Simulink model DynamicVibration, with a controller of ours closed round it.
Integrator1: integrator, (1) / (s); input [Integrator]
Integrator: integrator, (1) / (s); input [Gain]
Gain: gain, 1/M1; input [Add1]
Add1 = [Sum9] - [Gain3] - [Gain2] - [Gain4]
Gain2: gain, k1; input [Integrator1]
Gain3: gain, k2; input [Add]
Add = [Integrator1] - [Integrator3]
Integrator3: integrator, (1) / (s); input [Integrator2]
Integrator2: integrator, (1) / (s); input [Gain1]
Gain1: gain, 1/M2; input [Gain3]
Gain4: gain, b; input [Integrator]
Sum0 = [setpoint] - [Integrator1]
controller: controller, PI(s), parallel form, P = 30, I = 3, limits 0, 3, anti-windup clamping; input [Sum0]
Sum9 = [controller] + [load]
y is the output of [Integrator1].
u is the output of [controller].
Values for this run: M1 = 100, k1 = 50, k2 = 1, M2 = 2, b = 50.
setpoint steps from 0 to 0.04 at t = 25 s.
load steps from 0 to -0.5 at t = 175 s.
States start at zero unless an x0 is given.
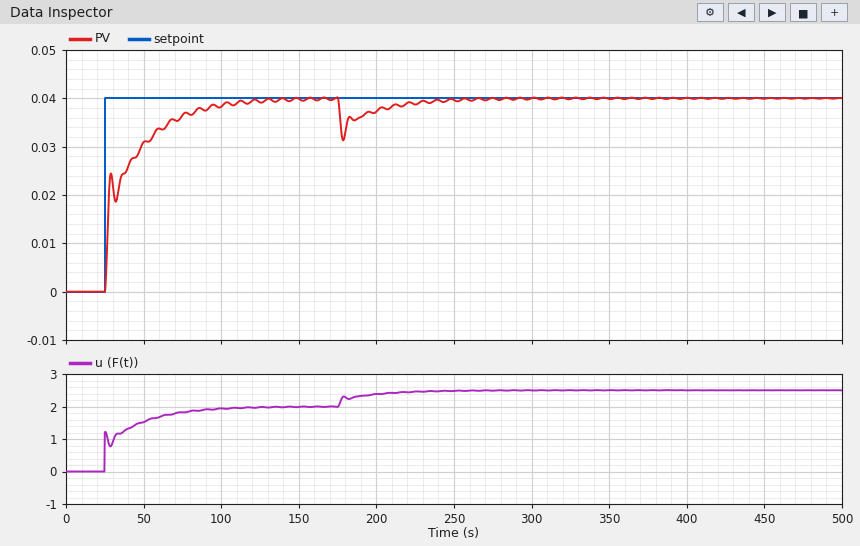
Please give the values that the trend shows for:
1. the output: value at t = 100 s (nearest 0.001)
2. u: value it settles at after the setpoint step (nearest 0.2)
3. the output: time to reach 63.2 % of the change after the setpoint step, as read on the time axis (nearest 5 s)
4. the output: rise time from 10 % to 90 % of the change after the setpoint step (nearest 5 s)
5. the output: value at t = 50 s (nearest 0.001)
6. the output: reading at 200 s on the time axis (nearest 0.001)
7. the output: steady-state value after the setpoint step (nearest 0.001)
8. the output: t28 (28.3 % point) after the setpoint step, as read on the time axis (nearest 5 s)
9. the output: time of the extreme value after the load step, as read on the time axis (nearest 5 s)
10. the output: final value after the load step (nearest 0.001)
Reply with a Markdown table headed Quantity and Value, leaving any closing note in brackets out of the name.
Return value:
| Quantity | Value |
|---|---|
| the output: value at t = 100 s | 0.038 |
| u: value it settles at after the setpoint step | 2.0 |
| the output: time to reach 63.2 % of the change after the setpoint step, as read on the time axis | 40 s |
| the output: rise time from 10 % to 90 % of the change after the setpoint step | 50 s |
| the output: value at t = 50 s | 0.031 |
| the output: reading at 200 s on the time axis | 0.037 |
| the output: steady-state value after the setpoint step | 0.040 |
| the output: t28 (28.3 % point) after the setpoint step, as read on the time axis | 25 s |
| the output: time of the extreme value after the load step, as read on the time axis | 180 s |
| the output: final value after the load step | 0.040 |
